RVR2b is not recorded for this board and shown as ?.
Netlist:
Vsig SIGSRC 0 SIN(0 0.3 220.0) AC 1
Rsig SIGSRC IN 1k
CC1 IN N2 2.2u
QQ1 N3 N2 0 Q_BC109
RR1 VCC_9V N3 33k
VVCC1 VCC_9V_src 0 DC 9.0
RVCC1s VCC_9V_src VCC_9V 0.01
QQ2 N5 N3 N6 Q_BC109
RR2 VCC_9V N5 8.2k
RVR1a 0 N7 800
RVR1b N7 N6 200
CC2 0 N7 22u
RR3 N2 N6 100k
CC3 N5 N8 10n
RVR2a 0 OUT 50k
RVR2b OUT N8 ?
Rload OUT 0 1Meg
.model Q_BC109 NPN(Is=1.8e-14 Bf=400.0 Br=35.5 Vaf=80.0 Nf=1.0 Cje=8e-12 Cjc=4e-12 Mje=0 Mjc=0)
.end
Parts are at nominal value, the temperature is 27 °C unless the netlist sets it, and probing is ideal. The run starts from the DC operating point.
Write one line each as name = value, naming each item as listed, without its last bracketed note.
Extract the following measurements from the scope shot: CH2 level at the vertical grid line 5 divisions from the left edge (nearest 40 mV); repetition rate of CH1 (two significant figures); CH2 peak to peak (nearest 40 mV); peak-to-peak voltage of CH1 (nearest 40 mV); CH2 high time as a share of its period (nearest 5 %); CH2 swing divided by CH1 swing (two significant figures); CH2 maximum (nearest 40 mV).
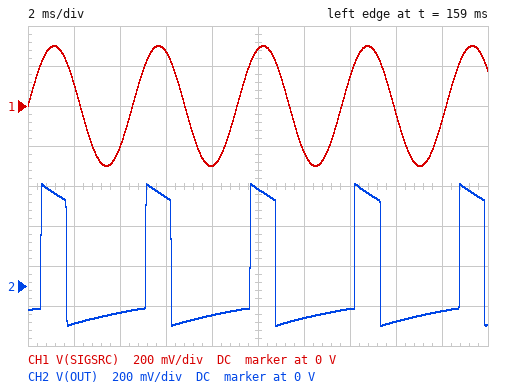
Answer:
CH2 level at the vertical grid line 5 divisions from the left edge = 480 mV
repetition rate of CH1 = 220 Hz
CH2 peak to peak = 720 mV
peak-to-peak voltage of CH1 = 600 mV
CH2 high time as a share of its period = 25 %
CH2 swing divided by CH1 swing = 1.2
CH2 maximum = 520 mV
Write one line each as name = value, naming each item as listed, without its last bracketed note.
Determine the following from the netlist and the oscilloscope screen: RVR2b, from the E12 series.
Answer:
RVR2b, from the E12 series = 560 kΩ
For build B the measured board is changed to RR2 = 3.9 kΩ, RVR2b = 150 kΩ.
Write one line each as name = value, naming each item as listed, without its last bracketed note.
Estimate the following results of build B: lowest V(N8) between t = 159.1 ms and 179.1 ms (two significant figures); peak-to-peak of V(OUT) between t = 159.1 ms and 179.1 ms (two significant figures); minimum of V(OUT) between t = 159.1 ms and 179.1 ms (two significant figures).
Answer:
lowest V(N8) between t = 159.1 ms and 179.1 ms = -4.1 V
peak-to-peak of V(OUT) between t = 159.1 ms and 179.1 ms = 2.5 V
minimum of V(OUT) between t = 159.1 ms and 179.1 ms = -980 mV
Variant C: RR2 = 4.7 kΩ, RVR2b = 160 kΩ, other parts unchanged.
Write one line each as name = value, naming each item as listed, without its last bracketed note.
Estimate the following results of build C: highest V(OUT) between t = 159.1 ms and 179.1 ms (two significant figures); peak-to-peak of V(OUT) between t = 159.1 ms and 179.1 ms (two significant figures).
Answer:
highest V(OUT) between t = 159.1 ms and 179.1 ms = 1.5 V
peak-to-peak of V(OUT) between t = 159.1 ms and 179.1 ms = 2.4 V
